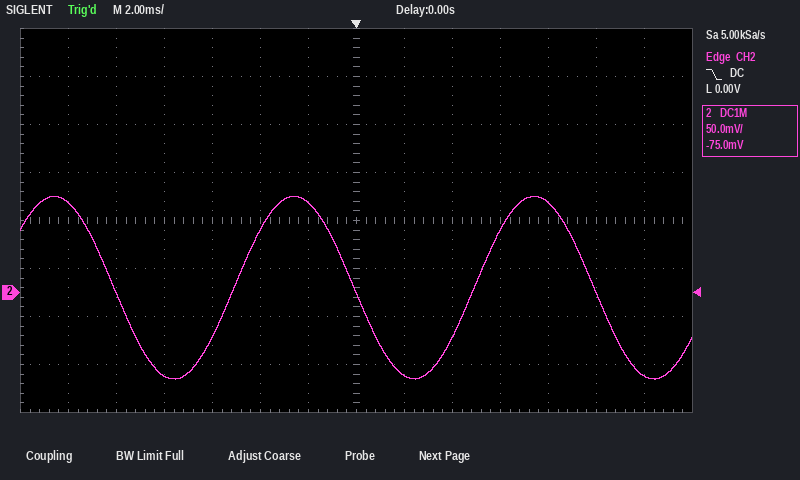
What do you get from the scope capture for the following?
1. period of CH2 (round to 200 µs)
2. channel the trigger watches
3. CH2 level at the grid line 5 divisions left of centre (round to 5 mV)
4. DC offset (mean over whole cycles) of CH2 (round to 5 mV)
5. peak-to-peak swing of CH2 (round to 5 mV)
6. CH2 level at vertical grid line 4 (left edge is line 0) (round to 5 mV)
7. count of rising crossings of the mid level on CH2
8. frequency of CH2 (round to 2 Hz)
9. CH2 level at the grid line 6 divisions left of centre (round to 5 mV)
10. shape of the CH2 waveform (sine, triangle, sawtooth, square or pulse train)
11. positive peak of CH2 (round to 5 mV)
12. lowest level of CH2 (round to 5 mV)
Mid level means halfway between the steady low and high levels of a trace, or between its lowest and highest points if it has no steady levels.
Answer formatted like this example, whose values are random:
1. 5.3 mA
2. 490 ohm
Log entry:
1. 10.0 ms
2. CH2
3. 0 mV
4. 5 mV
5. 190 mV
6. -45 mV
7. 2
8. 100 Hz
9. 95 mV
10. sine
11. 100 mV
12. -90 mV
